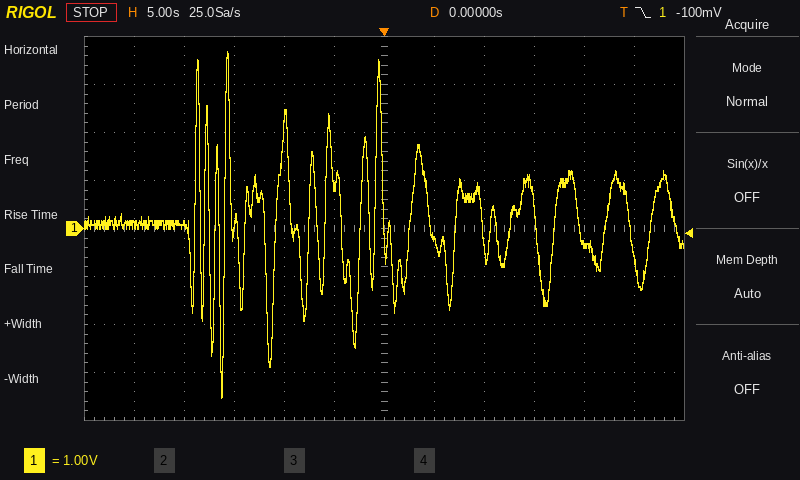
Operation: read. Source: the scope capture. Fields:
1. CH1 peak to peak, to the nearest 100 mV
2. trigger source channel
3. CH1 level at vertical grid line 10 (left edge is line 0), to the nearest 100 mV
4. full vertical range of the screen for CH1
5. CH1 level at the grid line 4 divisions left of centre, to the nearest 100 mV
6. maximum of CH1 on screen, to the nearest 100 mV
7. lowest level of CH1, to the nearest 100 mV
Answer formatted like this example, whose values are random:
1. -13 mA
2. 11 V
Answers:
1. 7.2 V
2. CH1
3. -300 mV
4. 8 V
5. 100 mV
6. 3.7 V
7. -3.5 V
